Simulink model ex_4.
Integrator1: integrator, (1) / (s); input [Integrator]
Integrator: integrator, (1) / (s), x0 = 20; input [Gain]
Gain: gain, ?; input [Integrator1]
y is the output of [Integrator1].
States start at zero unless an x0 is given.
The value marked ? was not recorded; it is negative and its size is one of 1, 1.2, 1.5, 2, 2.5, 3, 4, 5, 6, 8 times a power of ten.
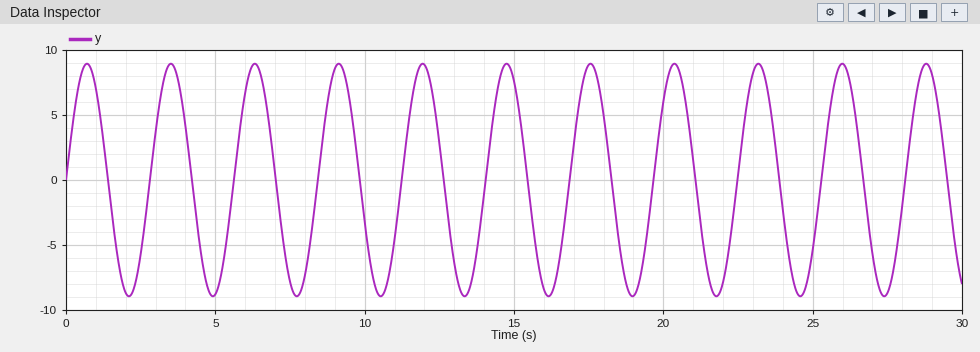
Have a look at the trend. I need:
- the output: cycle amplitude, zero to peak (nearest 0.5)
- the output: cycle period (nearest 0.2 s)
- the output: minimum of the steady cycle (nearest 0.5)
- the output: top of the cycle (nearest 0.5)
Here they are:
9.0
2.8 s
-9.0
9.0
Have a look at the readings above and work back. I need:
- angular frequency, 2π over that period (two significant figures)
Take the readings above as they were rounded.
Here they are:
2.2 rad/s
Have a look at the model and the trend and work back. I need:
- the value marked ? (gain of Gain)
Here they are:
-5
